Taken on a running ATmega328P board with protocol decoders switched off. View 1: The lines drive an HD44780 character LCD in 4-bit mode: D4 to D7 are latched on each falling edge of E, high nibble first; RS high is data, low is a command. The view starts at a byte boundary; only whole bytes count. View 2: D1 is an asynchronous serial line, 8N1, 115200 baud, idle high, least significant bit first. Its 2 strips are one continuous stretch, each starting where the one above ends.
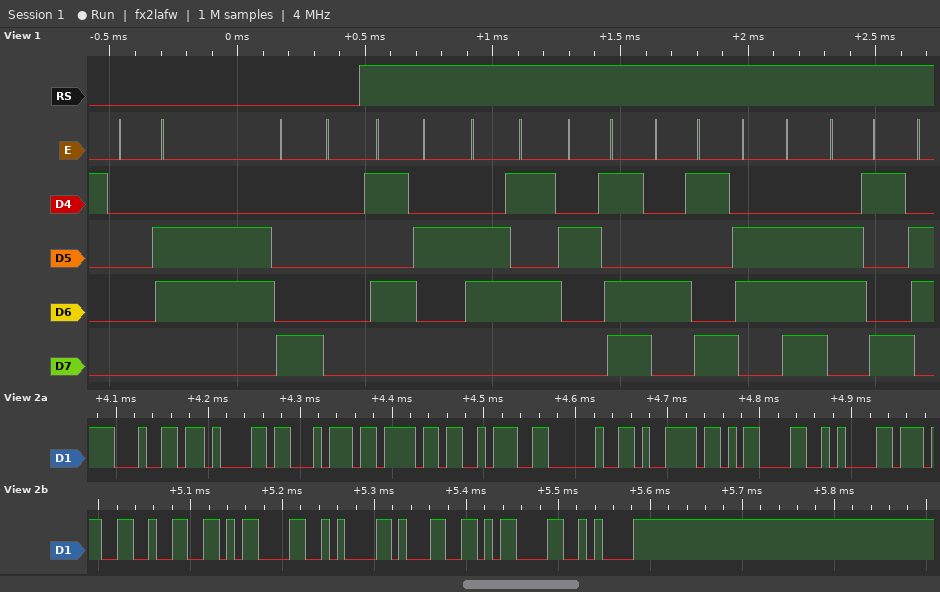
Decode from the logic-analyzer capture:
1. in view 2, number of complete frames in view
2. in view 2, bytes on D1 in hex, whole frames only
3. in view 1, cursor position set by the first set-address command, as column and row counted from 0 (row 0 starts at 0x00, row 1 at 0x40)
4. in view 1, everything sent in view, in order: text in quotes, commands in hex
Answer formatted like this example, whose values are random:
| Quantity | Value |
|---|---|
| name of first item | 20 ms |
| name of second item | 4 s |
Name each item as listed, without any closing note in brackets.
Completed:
| Quantity | Value |
|---|---|
| in view 2, number of complete frames in view | 16 |
| in view 2, bytes on D1 in hex, whole frames only | 64 61 74 6F 3A 20 79 0D 0A 37 32 0D 0A 31 0D 0A |
| in view 1, cursor position set by the first set-address command, as column and row counted from 0 | column 0, row 0 |
| in view 1, everything sent in view, in order: text in quotes, commands in hex | 0x06 0x80 "Re-Ini" |
